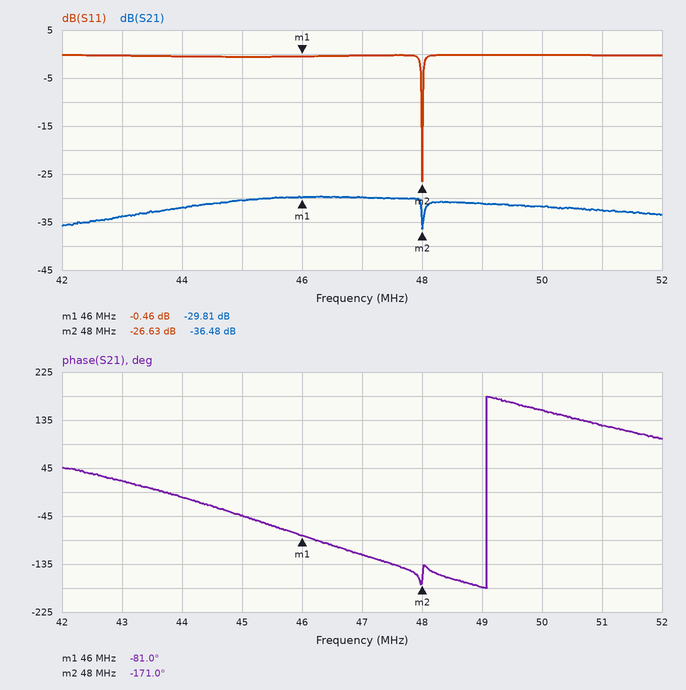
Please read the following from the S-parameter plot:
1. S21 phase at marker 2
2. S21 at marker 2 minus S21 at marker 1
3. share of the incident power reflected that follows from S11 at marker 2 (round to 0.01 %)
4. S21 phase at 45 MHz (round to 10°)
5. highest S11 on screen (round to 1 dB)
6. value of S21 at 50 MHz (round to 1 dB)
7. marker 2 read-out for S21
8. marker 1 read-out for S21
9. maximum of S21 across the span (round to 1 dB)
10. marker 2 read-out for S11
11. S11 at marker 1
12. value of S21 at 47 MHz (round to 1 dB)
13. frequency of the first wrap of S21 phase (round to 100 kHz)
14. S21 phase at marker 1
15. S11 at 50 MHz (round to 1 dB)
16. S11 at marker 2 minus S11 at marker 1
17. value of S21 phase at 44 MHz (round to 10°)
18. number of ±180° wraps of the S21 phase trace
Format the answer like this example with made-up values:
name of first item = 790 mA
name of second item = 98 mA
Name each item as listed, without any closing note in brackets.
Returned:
S21 phase at marker 2 = -171.0°
S21 at marker 2 minus S21 at marker 1 = -6.67 dB
share of the incident power reflected that follows from S11 at marker 2 = 0.22 %
S21 phase at 45 MHz = -40°
highest S11 on screen = 0 dB
value of S21 at 50 MHz = -32 dB
marker 2 read-out for S21 = -36.48 dB
marker 1 read-out for S21 = -29.81 dB
maximum of S21 across the span = -30 dB
marker 2 read-out for S11 = -26.63 dB
S11 at marker 1 = -0.46 dB
value of S21 at 47 MHz = -30 dB
frequency of the first wrap of S21 phase = 49.1 MHz
S21 phase at marker 1 = -81.0°
S11 at 50 MHz = 0 dB
S11 at marker 2 minus S11 at marker 1 = -26.17 dB
value of S21 phase at 44 MHz = -10°
number of ±180° wraps of the S21 phase trace = 1
